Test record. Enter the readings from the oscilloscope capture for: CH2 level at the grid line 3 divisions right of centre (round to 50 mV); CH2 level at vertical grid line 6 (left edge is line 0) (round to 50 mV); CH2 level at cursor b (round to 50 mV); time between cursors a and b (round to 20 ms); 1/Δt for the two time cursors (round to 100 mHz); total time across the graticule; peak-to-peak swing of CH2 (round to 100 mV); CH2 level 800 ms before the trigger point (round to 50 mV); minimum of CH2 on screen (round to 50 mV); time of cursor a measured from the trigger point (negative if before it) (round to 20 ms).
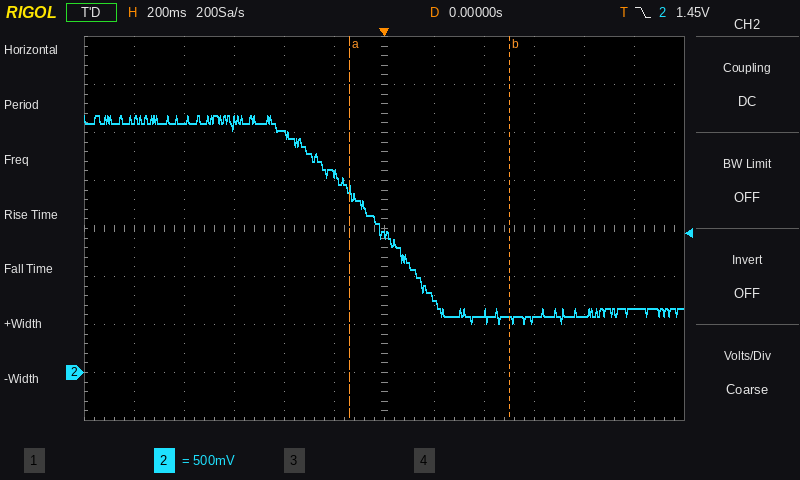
550 mV
1.45 V
550 mV
640 ms
1.6 Hz
2.4 s
2.20 V
2.60 V
500 mV
-140 ms
